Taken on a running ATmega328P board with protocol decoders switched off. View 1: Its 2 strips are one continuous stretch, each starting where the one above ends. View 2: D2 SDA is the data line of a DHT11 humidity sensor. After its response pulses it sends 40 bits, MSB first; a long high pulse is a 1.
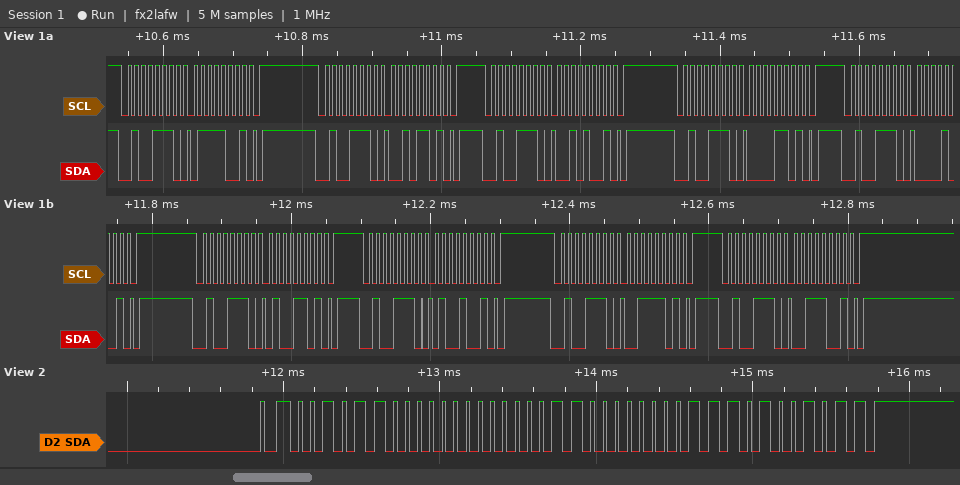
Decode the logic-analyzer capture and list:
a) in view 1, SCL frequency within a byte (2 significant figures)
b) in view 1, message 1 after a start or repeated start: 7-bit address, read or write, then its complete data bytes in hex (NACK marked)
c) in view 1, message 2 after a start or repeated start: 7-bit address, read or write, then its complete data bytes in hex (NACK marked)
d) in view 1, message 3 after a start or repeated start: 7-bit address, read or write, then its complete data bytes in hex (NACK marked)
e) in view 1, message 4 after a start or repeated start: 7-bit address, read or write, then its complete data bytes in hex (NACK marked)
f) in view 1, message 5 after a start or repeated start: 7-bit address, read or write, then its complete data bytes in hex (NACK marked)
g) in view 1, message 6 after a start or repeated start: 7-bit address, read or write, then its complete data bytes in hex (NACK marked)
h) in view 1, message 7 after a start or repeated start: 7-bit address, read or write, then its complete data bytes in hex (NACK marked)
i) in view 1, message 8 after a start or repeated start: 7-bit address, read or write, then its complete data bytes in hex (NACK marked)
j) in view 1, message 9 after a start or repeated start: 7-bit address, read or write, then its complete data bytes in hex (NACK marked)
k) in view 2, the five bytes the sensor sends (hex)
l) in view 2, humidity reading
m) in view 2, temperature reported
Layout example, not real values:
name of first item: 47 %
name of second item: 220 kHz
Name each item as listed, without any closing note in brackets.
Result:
in view 1, SCL frequency within a byte: 100 kHz
in view 1, message 1 after a start or repeated start: 7-bit address, read or write, then its complete data bytes in hex: 0x27 write: 79
in view 1, message 2 after a start or repeated start: 7-bit address, read or write, then its complete data bytes in hex: 0x27 write: 2D
in view 1, message 3 after a start or repeated start: 7-bit address, read or write, then its complete data bytes in hex: 0x27 write: 29
in view 1, message 4 after a start or repeated start: 7-bit address, read or write, then its complete data bytes in hex: 0x27 write: 0D
in view 1, message 5 after a start or repeated start: 7-bit address, read or write, then its complete data bytes in hex: 0x27 write: 09
in view 1, message 6 after a start or repeated start: 7-bit address, read or write, then its complete data bytes in hex: 0x27 write: 4D
in view 1, message 7 after a start or repeated start: 7-bit address, read or write, then its complete data bytes in hex: 0x27 write: 49
in view 1, message 8 after a start or repeated start: 7-bit address, read or write, then its complete data bytes in hex: 0x27 write: 3D
in view 1, message 9 after a start or repeated start: 7-bit address, read or write, then its complete data bytes in hex: 0x27 write: 39
in view 2, the five bytes the sensor sends: 2C 00 18 07 4B
in view 2, humidity reading: 44 %
in view 2, temperature reported: 24.7 °C
